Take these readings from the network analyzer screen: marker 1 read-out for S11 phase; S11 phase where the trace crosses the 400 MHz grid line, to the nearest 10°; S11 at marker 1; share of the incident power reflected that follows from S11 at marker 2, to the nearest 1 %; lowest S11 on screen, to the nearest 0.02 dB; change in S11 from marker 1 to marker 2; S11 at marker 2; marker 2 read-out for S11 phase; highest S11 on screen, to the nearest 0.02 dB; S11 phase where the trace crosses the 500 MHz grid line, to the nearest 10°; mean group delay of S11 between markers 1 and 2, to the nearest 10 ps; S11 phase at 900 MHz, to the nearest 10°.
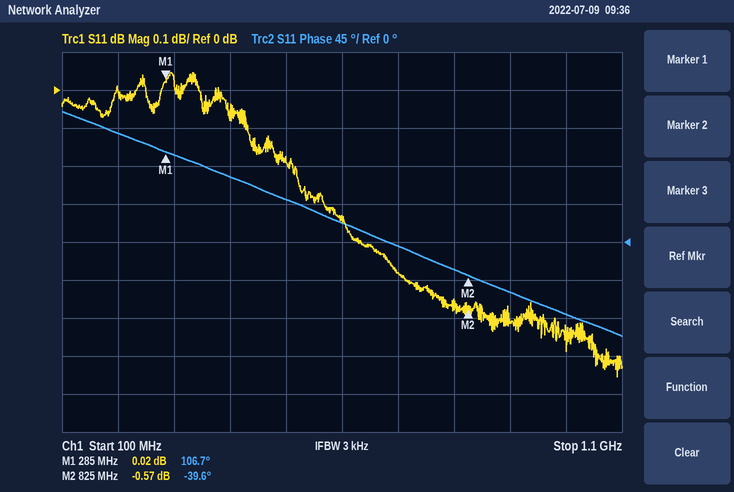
106.7°
80°
0.02 dB
88 %
-0.76 dB
-0.59 dB
-0.57 dB
-39.6°
0.04 dB
50°
750 ps
-60°
